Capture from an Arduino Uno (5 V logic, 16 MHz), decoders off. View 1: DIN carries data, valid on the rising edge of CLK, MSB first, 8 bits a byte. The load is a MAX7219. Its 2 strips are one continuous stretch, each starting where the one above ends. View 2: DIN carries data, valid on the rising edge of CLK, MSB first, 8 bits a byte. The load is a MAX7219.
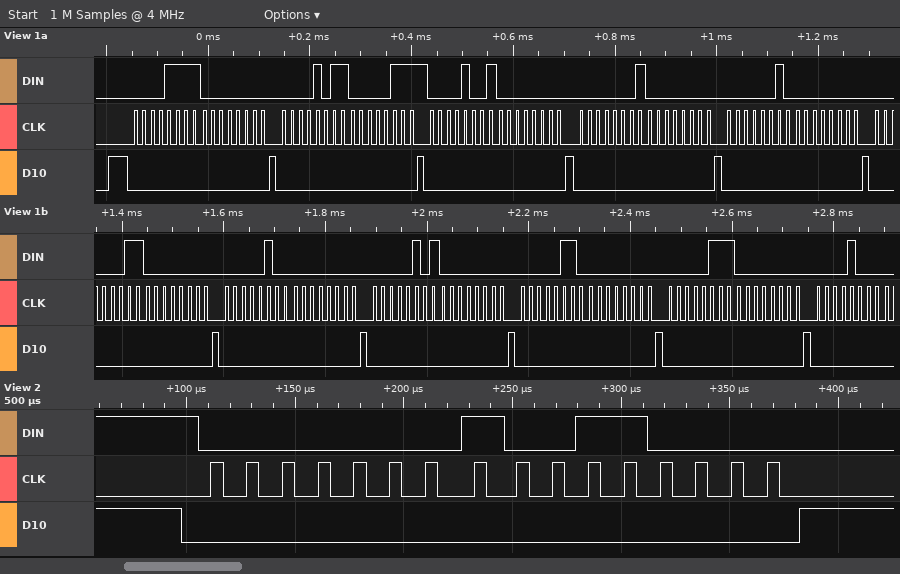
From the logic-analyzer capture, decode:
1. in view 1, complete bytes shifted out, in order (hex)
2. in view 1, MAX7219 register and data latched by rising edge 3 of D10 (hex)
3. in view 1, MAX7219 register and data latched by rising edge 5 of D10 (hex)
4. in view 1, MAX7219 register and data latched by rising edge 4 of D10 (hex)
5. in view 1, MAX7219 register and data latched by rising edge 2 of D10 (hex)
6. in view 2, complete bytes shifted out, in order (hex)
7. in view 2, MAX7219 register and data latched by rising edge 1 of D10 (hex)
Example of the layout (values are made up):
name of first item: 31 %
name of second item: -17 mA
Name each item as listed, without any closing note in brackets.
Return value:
in view 1, complete bytes shifted out, in order: 0F 00 0B 07 09 00 01 00 02 00 03 00 04 00 05 00 06 00 07 00 08
in view 1, MAX7219 register and data latched by rising edge 3 of D10: register 0xB, data 0x07
in view 1, MAX7219 register and data latched by rising edge 5 of D10: register 0x1, data 0x00
in view 1, MAX7219 register and data latched by rising edge 4 of D10: register 0x9, data 0x00
in view 1, MAX7219 register and data latched by rising edge 2 of D10: register 0xF, data 0x00
in view 2, complete bytes shifted out, in order: 0x01 0x30
in view 2, MAX7219 register and data latched by rising edge 1 of D10: register 0x1, data 0x30
